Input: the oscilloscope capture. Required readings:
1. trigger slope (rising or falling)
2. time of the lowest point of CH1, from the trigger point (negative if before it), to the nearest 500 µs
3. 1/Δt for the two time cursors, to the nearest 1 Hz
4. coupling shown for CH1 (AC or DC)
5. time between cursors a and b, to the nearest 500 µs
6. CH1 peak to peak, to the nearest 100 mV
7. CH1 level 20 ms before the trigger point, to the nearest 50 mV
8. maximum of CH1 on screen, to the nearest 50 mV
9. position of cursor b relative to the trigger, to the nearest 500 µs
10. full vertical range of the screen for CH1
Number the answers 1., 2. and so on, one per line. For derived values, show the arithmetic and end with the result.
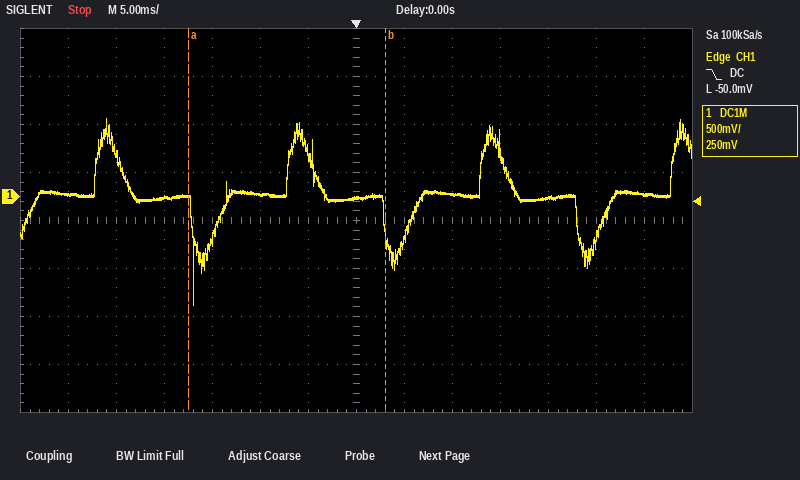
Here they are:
1. falling
2. -17.0 ms
3. 1 / 20.5 ms ≈ 49 Hz
4. DC
5. 20.5 ms
6. 1.90 V
7. 0 mV
8. 800 mV
9. +3.0 ms
10. 4 V
